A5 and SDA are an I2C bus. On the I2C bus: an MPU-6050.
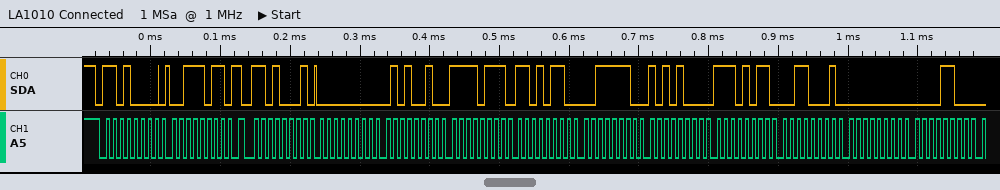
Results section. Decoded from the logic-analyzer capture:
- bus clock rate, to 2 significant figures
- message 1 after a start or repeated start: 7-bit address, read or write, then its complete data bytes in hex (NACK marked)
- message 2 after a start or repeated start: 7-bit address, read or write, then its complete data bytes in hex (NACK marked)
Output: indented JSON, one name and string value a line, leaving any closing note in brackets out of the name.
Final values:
{
  "bus clock rate, to 2 significant figures": "100 kHz",
  "message 1 after a start or repeated start: 7-bit address, read or write, then its complete data bytes in hex": "0x68 write: 3B",
  "message 2 after a start or repeated start: 7-bit address, read or write, then its complete data bytes in hex": "0x68 read: 00 52 F7 D6 3E A8 EB 31 00 0C"
}
